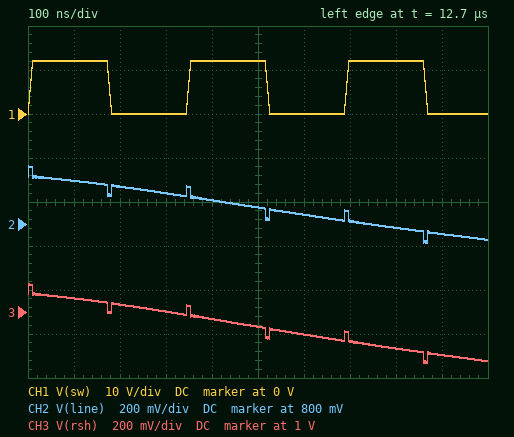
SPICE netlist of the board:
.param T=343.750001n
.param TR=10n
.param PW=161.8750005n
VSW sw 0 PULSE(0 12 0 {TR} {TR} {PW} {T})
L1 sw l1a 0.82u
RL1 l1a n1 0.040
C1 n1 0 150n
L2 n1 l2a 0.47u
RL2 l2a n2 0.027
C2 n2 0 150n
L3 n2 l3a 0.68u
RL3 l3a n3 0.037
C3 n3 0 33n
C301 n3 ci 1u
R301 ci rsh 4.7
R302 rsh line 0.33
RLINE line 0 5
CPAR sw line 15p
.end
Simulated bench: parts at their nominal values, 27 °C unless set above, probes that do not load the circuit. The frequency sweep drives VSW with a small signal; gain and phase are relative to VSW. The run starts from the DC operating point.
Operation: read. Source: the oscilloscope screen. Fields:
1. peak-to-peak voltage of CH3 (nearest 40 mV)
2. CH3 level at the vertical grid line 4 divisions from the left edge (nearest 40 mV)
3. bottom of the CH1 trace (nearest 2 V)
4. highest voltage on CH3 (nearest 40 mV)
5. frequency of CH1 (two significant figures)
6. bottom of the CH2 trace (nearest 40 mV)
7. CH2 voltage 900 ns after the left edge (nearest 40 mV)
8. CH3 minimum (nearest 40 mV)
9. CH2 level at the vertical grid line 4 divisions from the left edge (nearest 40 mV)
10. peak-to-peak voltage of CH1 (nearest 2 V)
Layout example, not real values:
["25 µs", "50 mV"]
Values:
["360 mV", "960 mV", "0 V", "1.12 V", "2.9 MHz", "720 mV", "760 mV", "760 mV", "920 mV", "12 V"]
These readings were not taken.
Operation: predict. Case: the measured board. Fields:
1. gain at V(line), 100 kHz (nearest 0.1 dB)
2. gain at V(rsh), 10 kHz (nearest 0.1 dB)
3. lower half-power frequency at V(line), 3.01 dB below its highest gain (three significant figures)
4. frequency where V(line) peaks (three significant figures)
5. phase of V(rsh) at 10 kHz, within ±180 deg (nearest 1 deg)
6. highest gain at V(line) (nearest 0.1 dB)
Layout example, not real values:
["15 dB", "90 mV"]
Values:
["-4.8 dB", "-10.9 dB", "236 kHz", "276 kHz", "57 deg", "6.6 dB"]
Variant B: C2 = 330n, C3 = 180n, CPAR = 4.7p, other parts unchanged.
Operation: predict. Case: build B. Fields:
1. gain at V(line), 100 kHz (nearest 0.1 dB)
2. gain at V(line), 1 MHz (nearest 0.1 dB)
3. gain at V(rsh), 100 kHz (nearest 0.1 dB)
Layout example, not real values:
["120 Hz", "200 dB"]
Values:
["-2.6 dB", "-35.0 dB", "-2.0 dB"]
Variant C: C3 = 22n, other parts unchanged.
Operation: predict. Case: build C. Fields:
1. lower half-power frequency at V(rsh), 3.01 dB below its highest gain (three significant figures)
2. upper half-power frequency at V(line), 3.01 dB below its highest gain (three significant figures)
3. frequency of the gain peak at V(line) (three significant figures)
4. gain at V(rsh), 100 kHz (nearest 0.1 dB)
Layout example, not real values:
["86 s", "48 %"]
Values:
["243 kHz", "322 kHz", "283 kHz", "-4.3 dB"]
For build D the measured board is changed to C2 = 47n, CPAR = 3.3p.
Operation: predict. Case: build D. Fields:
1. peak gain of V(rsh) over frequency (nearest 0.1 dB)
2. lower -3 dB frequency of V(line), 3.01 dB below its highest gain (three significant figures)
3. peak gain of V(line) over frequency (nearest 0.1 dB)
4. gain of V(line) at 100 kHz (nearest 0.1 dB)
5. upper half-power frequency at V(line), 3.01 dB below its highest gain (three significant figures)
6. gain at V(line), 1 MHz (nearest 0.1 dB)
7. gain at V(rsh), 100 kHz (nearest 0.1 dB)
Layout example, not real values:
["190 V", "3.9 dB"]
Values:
["6.0 dB", "289 kHz", "5.4 dB", "-5.3 dB", "411 kHz", "-11.5 dB", "-4.7 dB"]
